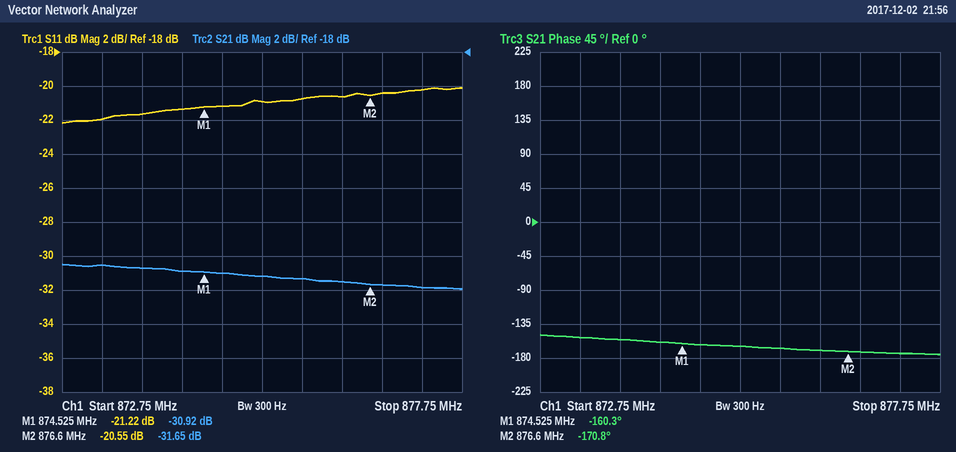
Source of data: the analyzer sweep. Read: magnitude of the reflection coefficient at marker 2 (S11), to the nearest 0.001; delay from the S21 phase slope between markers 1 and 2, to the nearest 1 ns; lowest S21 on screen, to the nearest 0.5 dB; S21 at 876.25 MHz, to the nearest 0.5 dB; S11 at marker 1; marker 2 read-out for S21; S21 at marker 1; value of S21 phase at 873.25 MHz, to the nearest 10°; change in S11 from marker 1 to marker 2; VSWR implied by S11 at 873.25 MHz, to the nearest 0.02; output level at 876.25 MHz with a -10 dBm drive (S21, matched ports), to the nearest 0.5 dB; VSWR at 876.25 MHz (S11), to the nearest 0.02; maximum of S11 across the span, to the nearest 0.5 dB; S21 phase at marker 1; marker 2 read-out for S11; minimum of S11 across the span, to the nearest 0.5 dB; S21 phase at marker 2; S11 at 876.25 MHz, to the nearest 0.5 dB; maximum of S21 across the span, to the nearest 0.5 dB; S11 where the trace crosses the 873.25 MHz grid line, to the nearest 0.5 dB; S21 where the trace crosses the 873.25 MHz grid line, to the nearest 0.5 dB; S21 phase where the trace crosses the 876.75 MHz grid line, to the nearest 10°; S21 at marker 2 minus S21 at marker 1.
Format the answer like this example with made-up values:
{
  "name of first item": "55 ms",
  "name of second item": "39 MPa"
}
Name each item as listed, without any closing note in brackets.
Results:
{
  "magnitude of the reflection coefficient at marker 2 (S11), to the nearest 0.001": "0.094",
  "delay from the S21 phase slope between markers 1 and 2, to the nearest 1 ns": "14 ns",
  "lowest S21 on screen, to the nearest 0.5 dB": "-32.0 dB",
  "S21 at 876.25 MHz, to the nearest 0.5 dB": "-31.5 dB",
  "S11 at marker 1": "-21.22 dB",
  "marker 2 read-out for S21": "-31.65 dB",
  "S21 at marker 1": "-30.92 dB",
  "value of S21 phase at 873.25 MHz, to the nearest 10°": "-150°",
  "change in S11 from marker 1 to marker 2": "0.67 dB",
  "VSWR implied by S11 at 873.25 MHz, to the nearest 0.02": "1.18",
  "output level at 876.25 MHz with a -10 dBm drive (S21, matched ports), to the nearest 0.5 dB": "-41.5 dBm",
  "VSWR at 876.25 MHz (S11), to the nearest 0.02": "1.20",
  "maximum of S11 across the span, to the nearest 0.5 dB": "-20.0 dB",
  "S21 phase at marker 1": "-160.3°",
  "marker 2 read-out for S11": "-20.55 dB",
  "minimum of S11 across the span, to the nearest 0.5 dB": "-22.0 dB",
  "S21 phase at marker 2": "-170.8°",
  "S11 at 876.25 MHz, to the nearest 0.5 dB": "-20.5 dB",
  "maximum of S21 across the span, to the nearest 0.5 dB": "-30.5 dB",
  "S11 where the trace crosses the 873.25 MHz grid line, to the nearest 0.5 dB": "-22.0 dB",
  "S21 where the trace crosses the 873.25 MHz grid line, to the nearest 0.5 dB": "-30.5 dB",
  "S21 phase where the trace crosses the 876.75 MHz grid line, to the nearest 10°": "-170°",
  "S21 at marker 2 minus S21 at marker 1": "-0.73 dB"
}
